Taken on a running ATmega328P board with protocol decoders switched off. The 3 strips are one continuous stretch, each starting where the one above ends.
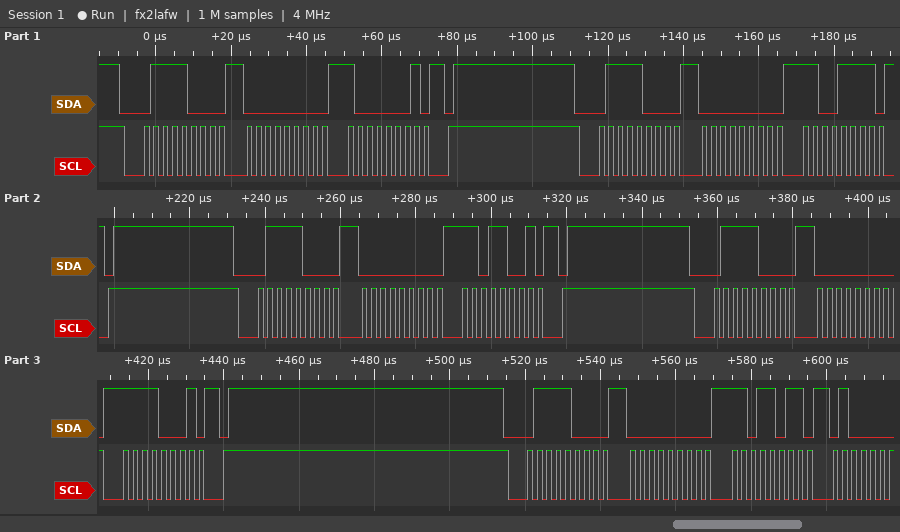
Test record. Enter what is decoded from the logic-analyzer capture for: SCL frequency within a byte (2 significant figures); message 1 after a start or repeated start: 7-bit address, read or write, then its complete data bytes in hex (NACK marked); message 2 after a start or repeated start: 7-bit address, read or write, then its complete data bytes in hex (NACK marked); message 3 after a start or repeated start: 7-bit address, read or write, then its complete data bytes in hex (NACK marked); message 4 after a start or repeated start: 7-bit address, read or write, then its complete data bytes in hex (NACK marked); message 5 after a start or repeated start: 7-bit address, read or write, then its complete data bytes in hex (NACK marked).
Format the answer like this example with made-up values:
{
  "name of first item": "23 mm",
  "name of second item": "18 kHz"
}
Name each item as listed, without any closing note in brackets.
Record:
{
  "SCL frequency within a byte": "400 kHz",
  "message 1 after a start or repeated start: 7-bit address, read or write, then its complete data bytes in hex": "0x3C write: 00 81",
  "message 2 after a start or repeated start: 7-bit address, read or write, then its complete data bytes in hex": "0x3C write: 00 CF",
  "message 3 after a start or repeated start: 7-bit address, read or write, then its complete data bytes in hex": "0x3C write: 00 D9",
  "message 4 after a start or repeated start: 7-bit address, read or write, then its complete data bytes in hex": "0x3C write: 00 F1",
  "message 5 after a start or repeated start: 7-bit address, read or write, then its complete data bytes in hex": "0x3C write: 00 DB"
}
